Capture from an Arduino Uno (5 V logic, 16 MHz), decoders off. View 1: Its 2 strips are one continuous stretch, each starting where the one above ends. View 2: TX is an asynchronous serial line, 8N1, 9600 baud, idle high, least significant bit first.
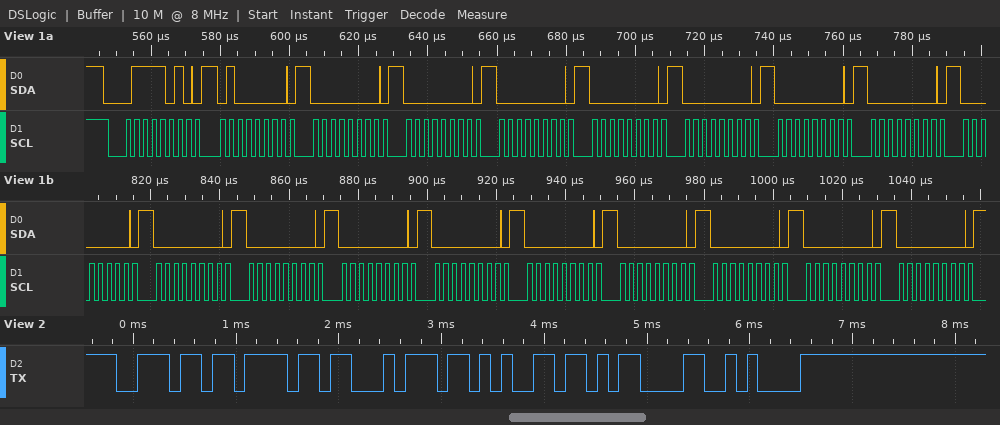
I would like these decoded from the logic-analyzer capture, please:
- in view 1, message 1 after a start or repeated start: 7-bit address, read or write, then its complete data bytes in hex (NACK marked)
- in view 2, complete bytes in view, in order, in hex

0x3D write: 40 00 00 00 00 00 00 00 00 00 00 00 00 00 00 00 00 00
0x6E 0x6F 0x74 0x65 0x0D 0x0A
